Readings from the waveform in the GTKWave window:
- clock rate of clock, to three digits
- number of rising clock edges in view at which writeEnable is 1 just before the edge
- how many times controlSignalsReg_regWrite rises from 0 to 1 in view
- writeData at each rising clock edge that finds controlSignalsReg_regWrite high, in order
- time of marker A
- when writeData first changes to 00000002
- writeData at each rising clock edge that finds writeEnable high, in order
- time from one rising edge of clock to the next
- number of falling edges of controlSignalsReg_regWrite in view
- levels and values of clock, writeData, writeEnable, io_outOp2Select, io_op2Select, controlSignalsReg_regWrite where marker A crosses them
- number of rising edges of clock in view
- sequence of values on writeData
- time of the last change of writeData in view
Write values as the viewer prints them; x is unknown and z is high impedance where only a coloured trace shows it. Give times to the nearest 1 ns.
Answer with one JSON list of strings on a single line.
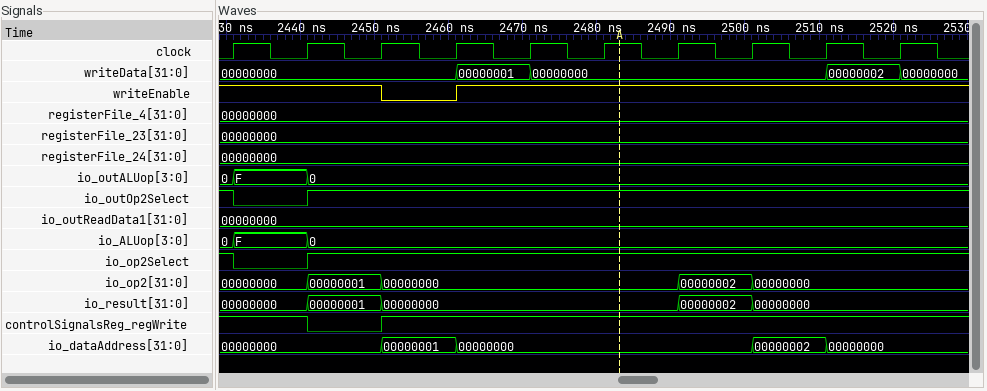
["100 MHz", "9", "1", "00000000, 00000000, 00000000, 00000001, 00000000, 00000000, 00000000, 00000000, 00000002", "2483 ns", "2511 ns", "00000000, 00000000, 00000000, 00000001, 00000000, 00000000, 00000000, 00000000, 00000002", "10 ns", "1", "clock=1, writeData=00000000, writeEnable=1, io_outOp2Select=1, io_op2Select=1, controlSignalsReg_regWrite=1", "10", "00000000, 00000001, 00000000, 00000002, 00000000", "2521 ns"]
